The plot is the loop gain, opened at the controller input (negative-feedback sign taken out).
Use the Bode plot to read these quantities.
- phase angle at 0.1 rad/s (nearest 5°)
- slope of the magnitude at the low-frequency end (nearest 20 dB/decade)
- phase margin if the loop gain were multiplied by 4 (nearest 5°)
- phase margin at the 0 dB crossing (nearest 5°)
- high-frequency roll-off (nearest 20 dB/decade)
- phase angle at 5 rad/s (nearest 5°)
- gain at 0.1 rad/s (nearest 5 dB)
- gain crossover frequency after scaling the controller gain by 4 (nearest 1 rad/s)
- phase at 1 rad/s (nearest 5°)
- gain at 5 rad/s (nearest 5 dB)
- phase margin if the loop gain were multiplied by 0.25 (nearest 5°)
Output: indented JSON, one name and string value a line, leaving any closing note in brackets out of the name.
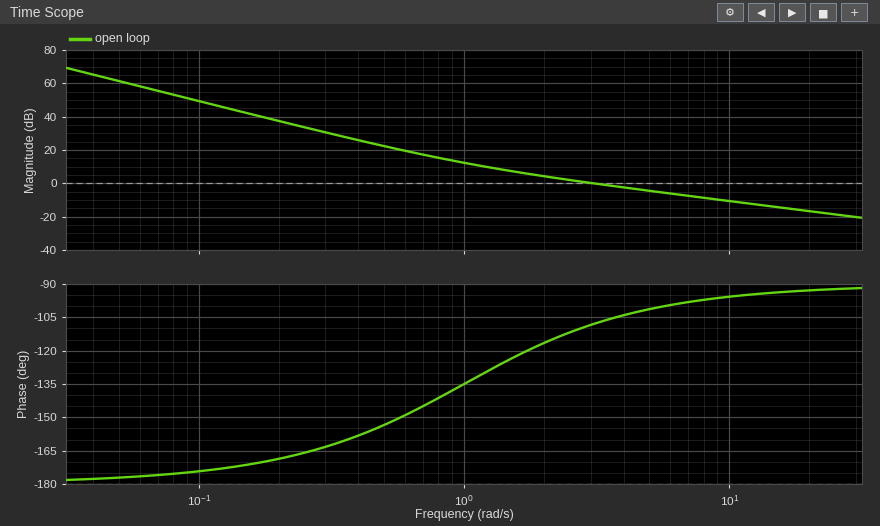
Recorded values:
{
  "phase angle at 0.1 rad/s": "-175°",
  "slope of the magnitude at the low-frequency end": "-40 dB/decade",
  "phase margin if the loop gain were multiplied by 4": "85°",
  "phase margin at the 0 dB crossing": "70°",
  "high-frequency roll-off": "-20 dB/decade",
  "phase angle at 5 rad/s": "-100°",
  "gain at 0.1 rad/s": "50 dB",
  "gain crossover frequency after scaling the controller gain by 4": "12 rad/s",
  "phase at 1 rad/s": "-135°",
  "gain at 5 rad/s": "-5 dB",
  "phase margin if the loop gain were multiplied by 0.25": "45°"
}
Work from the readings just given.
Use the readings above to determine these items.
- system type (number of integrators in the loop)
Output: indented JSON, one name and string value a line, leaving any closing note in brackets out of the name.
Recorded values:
{
  "system type": "2"
}
